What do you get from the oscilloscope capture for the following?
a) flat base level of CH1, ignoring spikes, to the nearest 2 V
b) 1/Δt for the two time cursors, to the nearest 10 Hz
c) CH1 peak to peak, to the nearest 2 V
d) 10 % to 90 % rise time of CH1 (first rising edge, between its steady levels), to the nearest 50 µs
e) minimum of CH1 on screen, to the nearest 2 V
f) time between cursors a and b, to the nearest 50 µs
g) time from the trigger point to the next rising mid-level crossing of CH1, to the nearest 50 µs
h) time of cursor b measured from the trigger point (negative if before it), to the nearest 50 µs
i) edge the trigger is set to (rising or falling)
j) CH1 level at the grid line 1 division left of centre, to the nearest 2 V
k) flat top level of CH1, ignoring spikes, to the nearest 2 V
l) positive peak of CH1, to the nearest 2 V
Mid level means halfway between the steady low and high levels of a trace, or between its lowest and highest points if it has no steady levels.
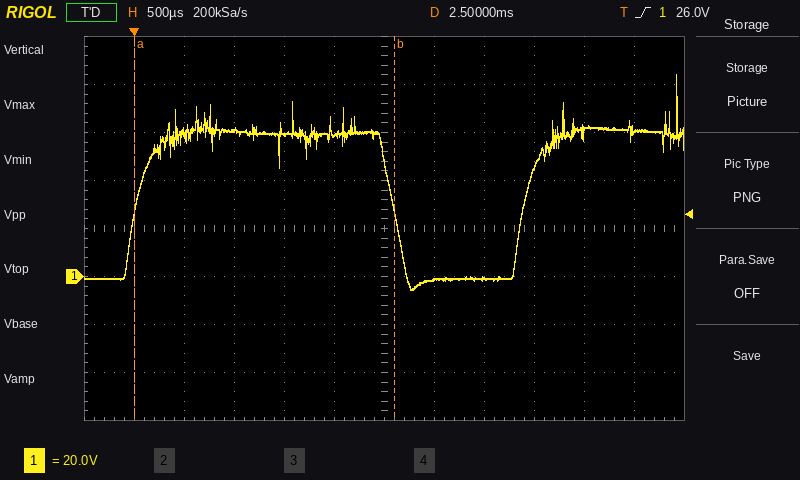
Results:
0 V
380 Hz
90 V
350 µs
-6 V
2.60 ms
3.90 ms
+2.60 ms
rising
60 V
60 V
84 V
